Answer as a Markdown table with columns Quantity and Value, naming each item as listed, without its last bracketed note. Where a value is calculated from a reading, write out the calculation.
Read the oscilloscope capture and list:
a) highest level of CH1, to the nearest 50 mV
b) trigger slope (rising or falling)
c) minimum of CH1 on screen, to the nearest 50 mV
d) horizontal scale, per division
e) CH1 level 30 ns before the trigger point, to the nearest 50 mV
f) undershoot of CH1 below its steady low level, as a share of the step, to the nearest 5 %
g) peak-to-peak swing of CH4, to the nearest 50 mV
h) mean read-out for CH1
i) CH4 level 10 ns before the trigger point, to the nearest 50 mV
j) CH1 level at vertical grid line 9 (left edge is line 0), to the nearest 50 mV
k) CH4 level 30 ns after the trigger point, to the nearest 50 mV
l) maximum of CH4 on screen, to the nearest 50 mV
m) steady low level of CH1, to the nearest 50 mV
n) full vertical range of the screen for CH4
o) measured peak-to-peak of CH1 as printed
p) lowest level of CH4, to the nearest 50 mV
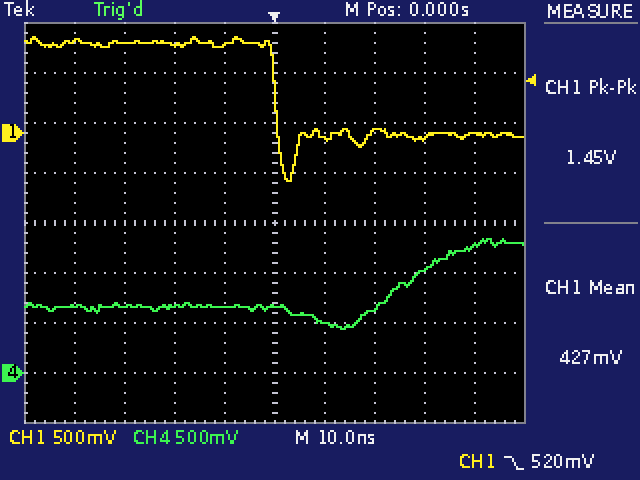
| Quantity | Value |
|---|---|
| highest level of CH1, to the nearest 50 mV | 950 mV |
| trigger slope | falling |
| minimum of CH1 on screen, to the nearest 50 mV | -500 mV |
| horizontal scale, per division | 10 ns |
| CH1 level 30 ns before the trigger point, to the nearest 50 mV | 900 mV |
| undershoot of CH1 below its steady low level, as a share of the step, to the nearest 5 % | 50 % |
| peak-to-peak swing of CH4, to the nearest 50 mV | 1.35 V − (450 mV) = 900 mV |
| mean read-out for CH1 | 427 mV |
| CH4 level 10 ns before the trigger point, to the nearest 50 mV | 650 mV |
| CH1 level at vertical grid line 9 (left edge is line 0), to the nearest 50 mV | 0 mV |
| CH4 level 30 ns after the trigger point, to the nearest 50 mV | 1.05 V |
| maximum of CH4 on screen, to the nearest 50 mV | 1.35 V |
| steady low level of CH1, to the nearest 50 mV | 0 mV |
| full vertical range of the screen for CH4 | 4 V |
| measured peak-to-peak of CH1 as printed | 1.45 V |
| lowest level of CH4, to the nearest 50 mV | 450 mV |
